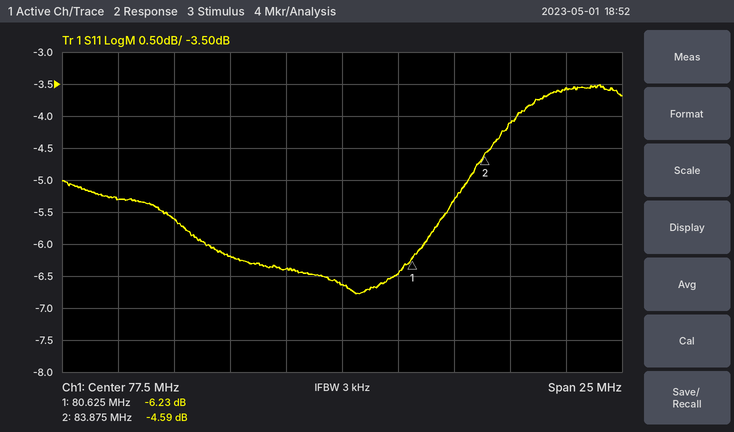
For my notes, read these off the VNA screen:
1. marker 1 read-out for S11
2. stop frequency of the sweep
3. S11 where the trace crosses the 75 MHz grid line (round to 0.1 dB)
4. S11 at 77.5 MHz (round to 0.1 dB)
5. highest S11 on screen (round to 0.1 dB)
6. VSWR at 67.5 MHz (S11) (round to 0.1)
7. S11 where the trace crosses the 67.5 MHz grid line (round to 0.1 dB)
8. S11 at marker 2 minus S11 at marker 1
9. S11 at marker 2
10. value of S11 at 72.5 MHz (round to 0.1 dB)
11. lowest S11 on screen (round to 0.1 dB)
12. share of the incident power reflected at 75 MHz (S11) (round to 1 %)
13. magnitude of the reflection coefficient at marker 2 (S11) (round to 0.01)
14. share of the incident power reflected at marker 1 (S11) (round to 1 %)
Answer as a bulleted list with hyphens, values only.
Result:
- -6.23 dB
- 90 MHz
- -6.4 dB
- -6.6 dB
- -3.5 dB
- 3.4
- -5.3 dB
- 1.64 dB
- -4.59 dB
- -6.2 dB
- -6.8 dB
- 23 %
- 0.59
- 24 %
